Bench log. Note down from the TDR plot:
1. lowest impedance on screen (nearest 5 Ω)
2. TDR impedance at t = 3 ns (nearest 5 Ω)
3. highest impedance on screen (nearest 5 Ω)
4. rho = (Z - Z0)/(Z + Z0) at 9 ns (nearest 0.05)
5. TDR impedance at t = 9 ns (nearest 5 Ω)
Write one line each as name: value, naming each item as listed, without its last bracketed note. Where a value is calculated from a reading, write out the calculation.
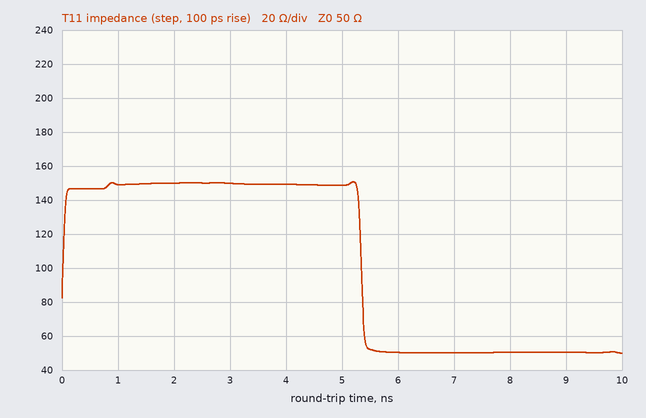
lowest impedance on screen: 50 Ω
TDR impedance at t = 3 ns: 150 Ω
highest impedance on screen: 150 Ω
rho = (Z - Z0)/(Z + Z0) at 9 ns: (50 − 50)/(50 + 50) ≈ 0.00
TDR impedance at t = 9 ns: 50 Ω
